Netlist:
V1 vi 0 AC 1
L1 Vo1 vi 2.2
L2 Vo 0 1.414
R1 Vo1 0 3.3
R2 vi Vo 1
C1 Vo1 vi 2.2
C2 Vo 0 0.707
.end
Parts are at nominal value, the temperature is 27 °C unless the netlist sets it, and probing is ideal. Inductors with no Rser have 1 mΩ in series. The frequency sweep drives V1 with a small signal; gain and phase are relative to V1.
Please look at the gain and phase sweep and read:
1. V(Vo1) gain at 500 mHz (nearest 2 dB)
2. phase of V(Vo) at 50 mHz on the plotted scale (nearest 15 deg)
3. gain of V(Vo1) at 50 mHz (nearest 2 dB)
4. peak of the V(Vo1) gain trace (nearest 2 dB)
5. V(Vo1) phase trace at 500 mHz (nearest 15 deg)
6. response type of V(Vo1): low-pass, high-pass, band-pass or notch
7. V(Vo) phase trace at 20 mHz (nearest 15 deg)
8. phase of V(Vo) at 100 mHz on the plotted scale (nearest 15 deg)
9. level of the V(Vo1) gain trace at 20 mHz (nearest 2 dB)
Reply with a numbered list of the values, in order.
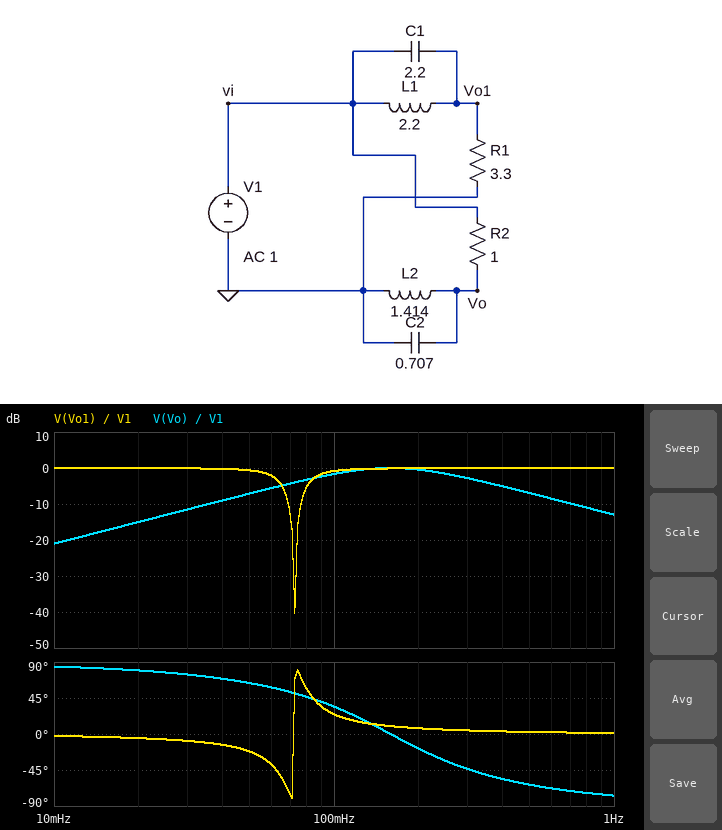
1. 0 dB
2. 60 deg
3. 0 dB
4. 0 dB
5. 0 deg
6. notch
7. 75 deg
8. 30 deg
9. 0 dB
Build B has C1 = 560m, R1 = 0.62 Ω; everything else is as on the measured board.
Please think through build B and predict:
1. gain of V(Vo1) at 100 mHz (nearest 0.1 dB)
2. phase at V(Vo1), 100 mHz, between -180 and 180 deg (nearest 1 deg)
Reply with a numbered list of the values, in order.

1. -13.0 dB
2. -77 deg
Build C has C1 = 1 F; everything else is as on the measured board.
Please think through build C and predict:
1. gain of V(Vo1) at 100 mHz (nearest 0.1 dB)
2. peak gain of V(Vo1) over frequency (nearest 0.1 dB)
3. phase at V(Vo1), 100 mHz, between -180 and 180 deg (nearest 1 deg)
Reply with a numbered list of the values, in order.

1. -10.5 dB
2. 0 dB
3. -72 deg
